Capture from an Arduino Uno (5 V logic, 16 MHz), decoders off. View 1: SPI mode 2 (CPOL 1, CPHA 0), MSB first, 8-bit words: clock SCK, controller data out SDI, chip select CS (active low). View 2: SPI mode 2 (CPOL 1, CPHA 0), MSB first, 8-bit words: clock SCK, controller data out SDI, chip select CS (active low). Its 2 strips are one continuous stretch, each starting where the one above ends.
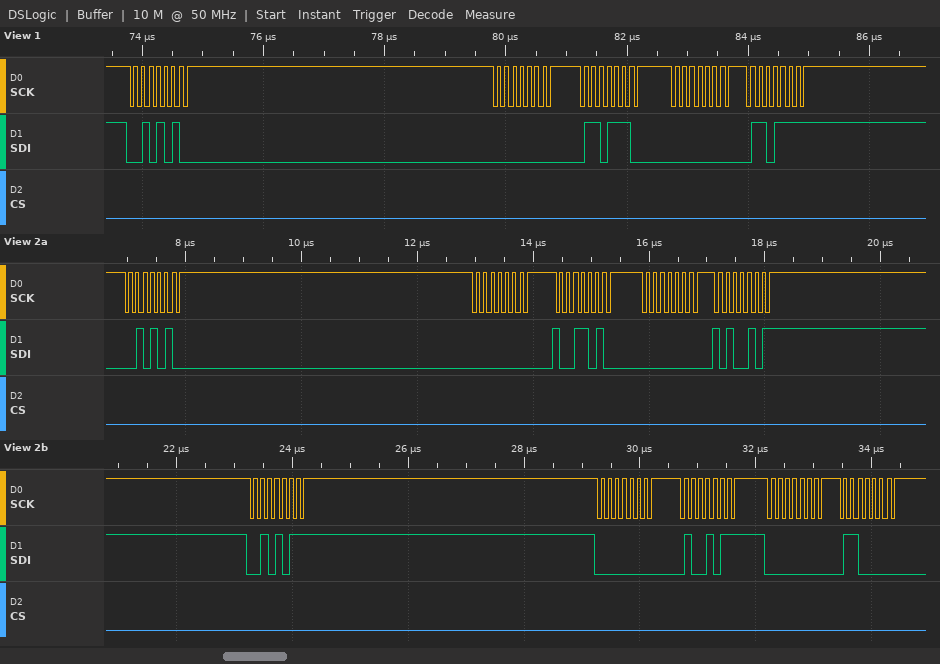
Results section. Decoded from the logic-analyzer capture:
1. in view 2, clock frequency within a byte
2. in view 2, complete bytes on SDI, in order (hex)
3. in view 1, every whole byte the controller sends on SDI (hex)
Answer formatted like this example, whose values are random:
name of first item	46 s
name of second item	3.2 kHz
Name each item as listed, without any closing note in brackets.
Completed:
in view 2, clock frequency within a byte	8 MHz
in view 2, complete bytes on SDI, in order	2A 00 9A 00 A5 2B 00 4B 00 60
in view 1, every whole byte the controller sends on SDI	2A 00 6E 00 6F
